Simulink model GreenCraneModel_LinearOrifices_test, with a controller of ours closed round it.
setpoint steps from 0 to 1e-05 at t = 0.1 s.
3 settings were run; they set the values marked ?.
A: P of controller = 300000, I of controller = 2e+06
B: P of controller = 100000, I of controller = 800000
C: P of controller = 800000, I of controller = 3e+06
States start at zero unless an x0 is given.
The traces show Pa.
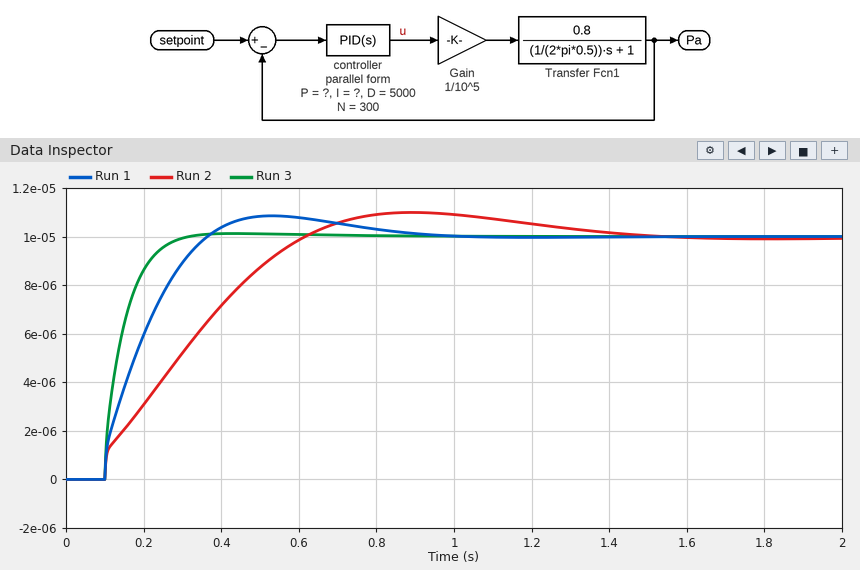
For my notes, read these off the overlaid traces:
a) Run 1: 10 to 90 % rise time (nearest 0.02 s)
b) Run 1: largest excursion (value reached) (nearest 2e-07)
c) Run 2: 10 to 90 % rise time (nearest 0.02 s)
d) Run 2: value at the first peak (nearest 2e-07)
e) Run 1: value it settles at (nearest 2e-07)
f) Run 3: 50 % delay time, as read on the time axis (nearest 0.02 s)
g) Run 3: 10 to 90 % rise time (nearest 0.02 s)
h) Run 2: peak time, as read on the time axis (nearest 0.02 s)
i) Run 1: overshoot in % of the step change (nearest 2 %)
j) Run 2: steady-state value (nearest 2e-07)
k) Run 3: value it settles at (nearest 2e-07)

0.20 s
0.0000108
0.42 s
0.0000110
0.0000100
0.14 s
0.12 s
0.90 s
8 %
0.0000100
0.0000100
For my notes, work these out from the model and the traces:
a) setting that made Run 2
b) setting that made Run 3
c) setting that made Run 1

B
C
A
